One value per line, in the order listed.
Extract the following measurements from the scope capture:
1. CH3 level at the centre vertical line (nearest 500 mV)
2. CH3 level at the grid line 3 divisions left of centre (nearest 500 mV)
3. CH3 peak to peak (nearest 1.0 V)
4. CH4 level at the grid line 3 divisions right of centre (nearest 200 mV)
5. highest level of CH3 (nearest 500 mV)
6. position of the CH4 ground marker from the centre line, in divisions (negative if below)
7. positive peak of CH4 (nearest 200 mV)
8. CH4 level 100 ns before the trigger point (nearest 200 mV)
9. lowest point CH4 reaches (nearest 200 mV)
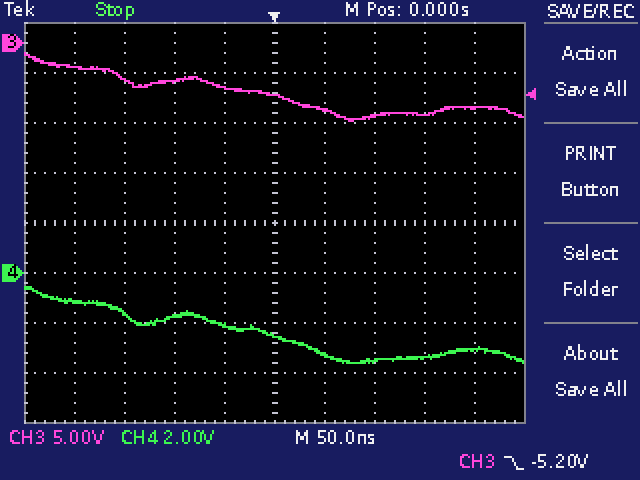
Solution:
-5.0 V
-3.5 V
7.0 V
-3.4 V
-1.0 V
-1.0 div
-600 mV
-1.8 V
-3.6 V
